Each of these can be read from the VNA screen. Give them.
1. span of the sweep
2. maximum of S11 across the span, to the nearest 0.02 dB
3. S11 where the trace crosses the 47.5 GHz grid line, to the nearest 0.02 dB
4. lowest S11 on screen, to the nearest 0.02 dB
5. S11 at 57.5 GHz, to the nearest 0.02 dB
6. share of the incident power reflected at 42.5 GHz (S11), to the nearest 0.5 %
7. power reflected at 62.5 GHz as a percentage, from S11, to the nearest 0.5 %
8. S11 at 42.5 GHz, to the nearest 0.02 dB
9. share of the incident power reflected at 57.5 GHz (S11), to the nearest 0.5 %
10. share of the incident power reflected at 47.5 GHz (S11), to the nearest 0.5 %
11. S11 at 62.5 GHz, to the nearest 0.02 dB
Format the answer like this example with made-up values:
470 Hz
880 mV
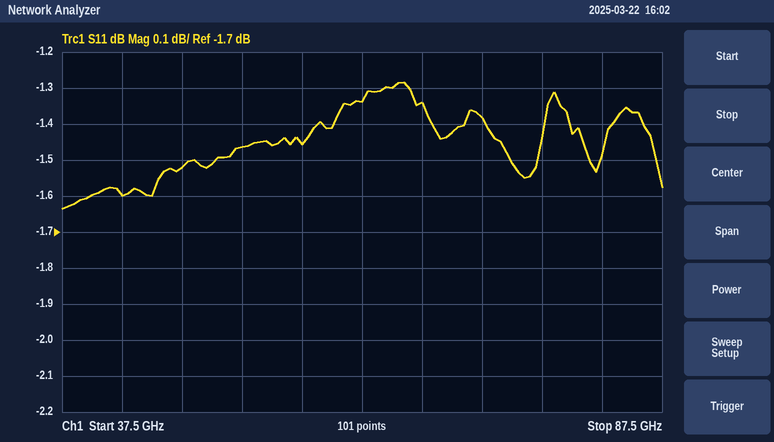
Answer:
50 GHz
-1.28 dB
-1.52 dB
-1.64 dB
-1.46 dB
69.0 %
73.5 %
-1.60 dB
71.5 %
70.5 %
-1.34 dB
